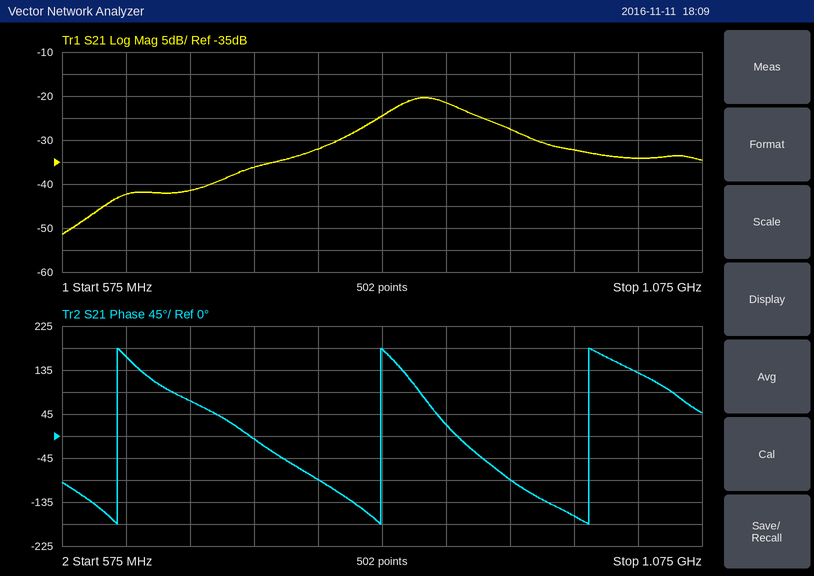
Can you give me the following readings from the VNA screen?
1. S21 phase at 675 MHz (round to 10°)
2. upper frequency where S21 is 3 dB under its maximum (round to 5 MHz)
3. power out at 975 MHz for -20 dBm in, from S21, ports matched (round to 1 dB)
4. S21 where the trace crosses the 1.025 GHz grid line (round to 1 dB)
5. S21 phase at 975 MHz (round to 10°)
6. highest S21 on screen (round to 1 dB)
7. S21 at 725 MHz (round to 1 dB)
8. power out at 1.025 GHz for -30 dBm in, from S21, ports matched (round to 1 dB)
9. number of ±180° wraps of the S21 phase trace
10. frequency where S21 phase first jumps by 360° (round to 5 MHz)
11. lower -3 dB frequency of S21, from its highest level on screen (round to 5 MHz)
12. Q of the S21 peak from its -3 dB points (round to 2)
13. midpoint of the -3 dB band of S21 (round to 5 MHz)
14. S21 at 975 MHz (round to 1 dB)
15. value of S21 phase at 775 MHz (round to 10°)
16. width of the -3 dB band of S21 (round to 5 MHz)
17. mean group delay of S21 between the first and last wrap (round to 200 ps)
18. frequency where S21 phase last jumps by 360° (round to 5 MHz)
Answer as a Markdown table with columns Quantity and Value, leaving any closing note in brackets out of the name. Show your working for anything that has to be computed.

| Quantity | Value |
|---|---|
| S21 phase at 675 MHz | 70° |
| upper frequency where S21 is 3 dB under its maximum | 890 MHz |
| power out at 975 MHz for -20 dBm in, from S21, ports matched | -20 dBm + (-32 dB) = -52 dBm |
| S21 where the trace crosses the 1.025 GHz grid line | -34 dB |
| S21 phase at 975 MHz | -160° |
| highest S21 on screen | -20 dB |
| S21 at 725 MHz | -36 dB |
| power out at 1.025 GHz for -30 dBm in, from S21, ports matched | -30 dBm + (-34 dB) = -64 dBm |
| number of ±180° wraps of the S21 phase trace | 3 |
| frequency where S21 phase first jumps by 360° | 620 MHz |
| lower -3 dB frequency of S21, from its highest level on screen | 830 MHz |
| Q of the S21 peak from its -3 dB points | 860 MHz / 60 MHz ≈ 14 |
| midpoint of the -3 dB band of S21 | 860 MHz |
| S21 at 975 MHz | -32 dB |
| value of S21 phase at 775 MHz | -90° |
| width of the -3 dB band of S21 | 890 MHz − 830 MHz = 60 MHz |
| mean group delay of S21 between the first and last wrap | 2 cycles / (985 MHz − 620 MHz) ≈ 5.48 ns, so 5.4 ns to the nearest 200 ps |
| frequency where S21 phase last jumps by 360° | 985 MHz |
